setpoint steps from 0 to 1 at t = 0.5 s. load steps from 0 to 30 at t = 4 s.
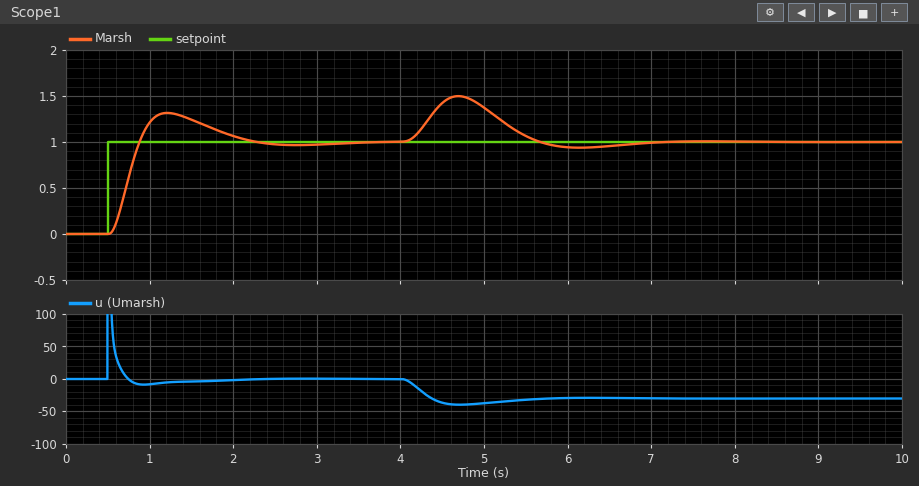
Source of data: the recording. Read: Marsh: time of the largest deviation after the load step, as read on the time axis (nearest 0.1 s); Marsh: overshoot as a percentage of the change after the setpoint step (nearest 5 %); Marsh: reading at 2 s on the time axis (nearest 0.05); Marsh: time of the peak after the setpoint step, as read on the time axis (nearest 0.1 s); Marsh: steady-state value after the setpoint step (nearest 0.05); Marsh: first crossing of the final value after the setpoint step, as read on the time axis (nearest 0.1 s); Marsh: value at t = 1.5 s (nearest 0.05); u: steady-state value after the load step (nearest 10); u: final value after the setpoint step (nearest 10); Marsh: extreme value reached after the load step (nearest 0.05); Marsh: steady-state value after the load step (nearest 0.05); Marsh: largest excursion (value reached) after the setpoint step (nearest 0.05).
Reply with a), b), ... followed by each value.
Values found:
a) 4.7 s
b) 30 %
c) 1.05
d) 1.2 s
e) 1.00
f) 0.9 s
g) 1.25
h) -30
i) 0
j) 1.50
k) 1.00
l) 1.30
